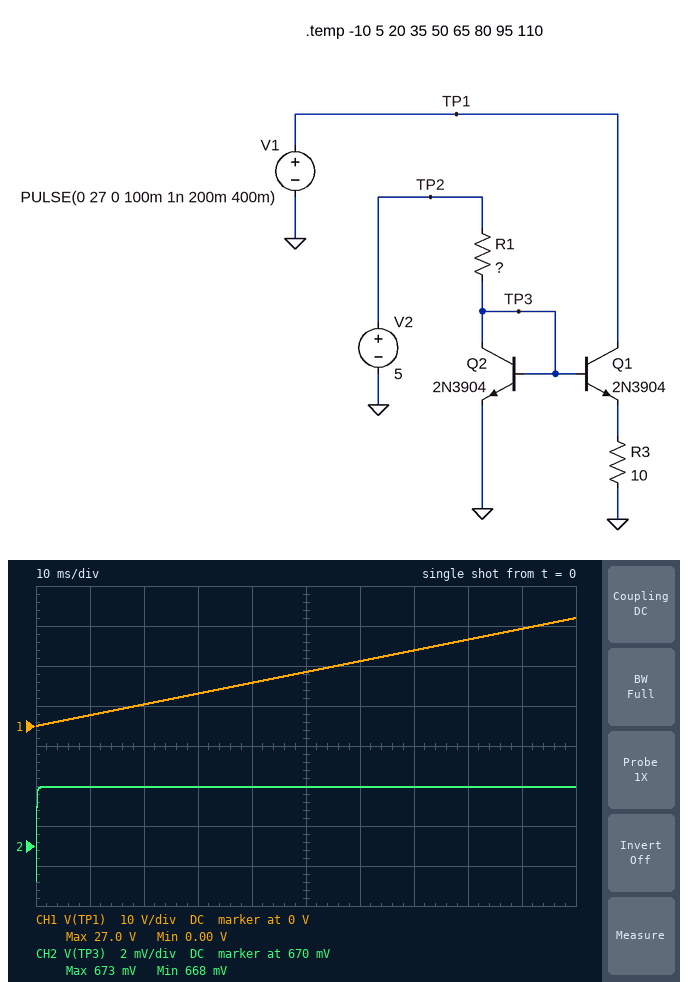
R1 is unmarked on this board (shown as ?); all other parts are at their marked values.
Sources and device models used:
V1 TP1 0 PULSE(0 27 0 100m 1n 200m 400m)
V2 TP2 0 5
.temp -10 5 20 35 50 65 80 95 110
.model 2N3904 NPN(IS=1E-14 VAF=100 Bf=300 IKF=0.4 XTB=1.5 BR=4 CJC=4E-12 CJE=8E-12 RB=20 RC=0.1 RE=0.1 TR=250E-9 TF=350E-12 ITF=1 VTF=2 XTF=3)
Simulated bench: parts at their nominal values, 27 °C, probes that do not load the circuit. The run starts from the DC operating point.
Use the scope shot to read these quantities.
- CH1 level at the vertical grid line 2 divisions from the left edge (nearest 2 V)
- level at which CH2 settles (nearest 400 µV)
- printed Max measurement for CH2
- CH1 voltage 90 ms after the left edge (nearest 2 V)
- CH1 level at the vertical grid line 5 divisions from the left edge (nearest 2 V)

6 V
672.8 mV
673 mV
24 V
14 V
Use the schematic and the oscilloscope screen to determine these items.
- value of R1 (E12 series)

2.2 kΩ
